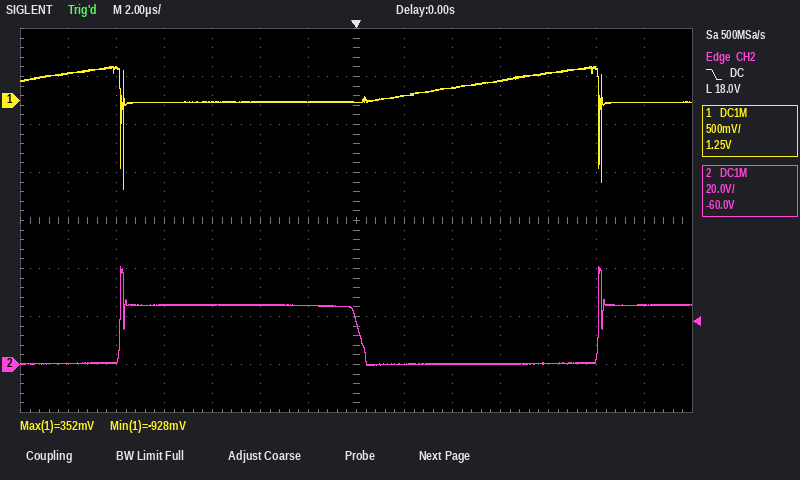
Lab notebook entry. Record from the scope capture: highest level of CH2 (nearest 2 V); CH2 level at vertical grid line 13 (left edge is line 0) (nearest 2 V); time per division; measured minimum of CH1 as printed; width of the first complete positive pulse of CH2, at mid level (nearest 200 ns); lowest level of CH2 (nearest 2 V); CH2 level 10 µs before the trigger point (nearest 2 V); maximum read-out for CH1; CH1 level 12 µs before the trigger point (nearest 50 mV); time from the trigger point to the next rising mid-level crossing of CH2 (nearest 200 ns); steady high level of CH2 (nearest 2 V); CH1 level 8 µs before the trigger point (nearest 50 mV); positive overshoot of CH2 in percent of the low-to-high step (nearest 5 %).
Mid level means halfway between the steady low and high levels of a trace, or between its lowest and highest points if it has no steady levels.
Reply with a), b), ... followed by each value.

a) 40 V
b) 24 V
c) 2 µs
d) -928 mV
e) 10.0 µs
f) 0 V
g) 2 V
h) 352 mV
i) 300 mV
j) 10.0 µs
k) 24 V
l) 0 mV
m) 65 %
